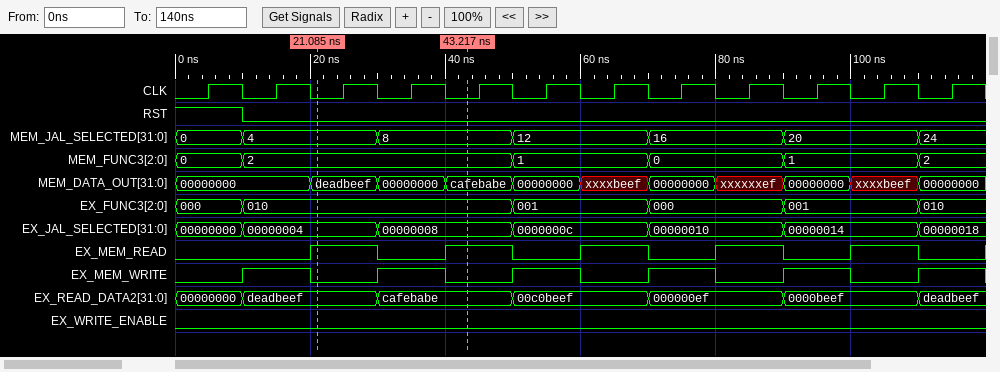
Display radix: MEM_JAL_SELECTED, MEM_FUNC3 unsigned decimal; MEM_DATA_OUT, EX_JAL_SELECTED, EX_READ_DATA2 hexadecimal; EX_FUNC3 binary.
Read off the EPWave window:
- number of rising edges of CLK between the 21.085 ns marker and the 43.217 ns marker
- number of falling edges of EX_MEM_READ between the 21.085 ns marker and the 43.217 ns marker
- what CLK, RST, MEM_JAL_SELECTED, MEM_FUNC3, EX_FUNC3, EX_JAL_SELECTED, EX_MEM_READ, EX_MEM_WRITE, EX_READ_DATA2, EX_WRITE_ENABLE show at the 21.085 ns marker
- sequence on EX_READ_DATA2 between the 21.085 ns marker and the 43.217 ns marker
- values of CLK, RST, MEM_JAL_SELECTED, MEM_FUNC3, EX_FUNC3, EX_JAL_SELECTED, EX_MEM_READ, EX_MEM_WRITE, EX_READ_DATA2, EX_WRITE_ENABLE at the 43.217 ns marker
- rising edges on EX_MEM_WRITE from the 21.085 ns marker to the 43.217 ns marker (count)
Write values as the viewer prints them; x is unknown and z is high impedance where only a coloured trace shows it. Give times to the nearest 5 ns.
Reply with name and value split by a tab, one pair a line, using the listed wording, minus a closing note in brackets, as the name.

number of rising edges of CLK between the 21.085 ns marker and the 43.217 ns marker	2
number of falling edges of EX_MEM_READ between the 21.085 ns marker and the 43.217 ns marker	1
what CLK, RST, MEM_JAL_SELECTED, MEM_FUNC3, EX_FUNC3, EX_JAL_SELECTED, EX_MEM_READ, EX_MEM_WRITE, EX_READ_DATA2, EX_WRITE_ENABLE show at the 21.085 ns marker	CLK=0, RST=0, MEM_JAL_SELECTED=4, MEM_FUNC3=2, EX_FUNC3=010, EX_JAL_SELECTED=00000004, EX_MEM_READ=1, EX_MEM_WRITE=0, EX_READ_DATA2=deadbeef, EX_WRITE_ENABLE=0
sequence on EX_READ_DATA2 between the 21.085 ns marker and the 43.217 ns marker	deadbeef, cafebabe
values of CLK, RST, MEM_JAL_SELECTED, MEM_FUNC3, EX_FUNC3, EX_JAL_SELECTED, EX_MEM_READ, EX_MEM_WRITE, EX_READ_DATA2, EX_WRITE_ENABLE at the 43.217 ns marker	CLK=0, RST=0, MEM_JAL_SELECTED=8, MEM_FUNC3=2, EX_FUNC3=010, EX_JAL_SELECTED=00000008, EX_MEM_READ=1, EX_MEM_WRITE=0, EX_READ_DATA2=cafebabe, EX_WRITE_ENABLE=0
rising edges on EX_MEM_WRITE from the 21.085 ns marker to the 43.217 ns marker	1
